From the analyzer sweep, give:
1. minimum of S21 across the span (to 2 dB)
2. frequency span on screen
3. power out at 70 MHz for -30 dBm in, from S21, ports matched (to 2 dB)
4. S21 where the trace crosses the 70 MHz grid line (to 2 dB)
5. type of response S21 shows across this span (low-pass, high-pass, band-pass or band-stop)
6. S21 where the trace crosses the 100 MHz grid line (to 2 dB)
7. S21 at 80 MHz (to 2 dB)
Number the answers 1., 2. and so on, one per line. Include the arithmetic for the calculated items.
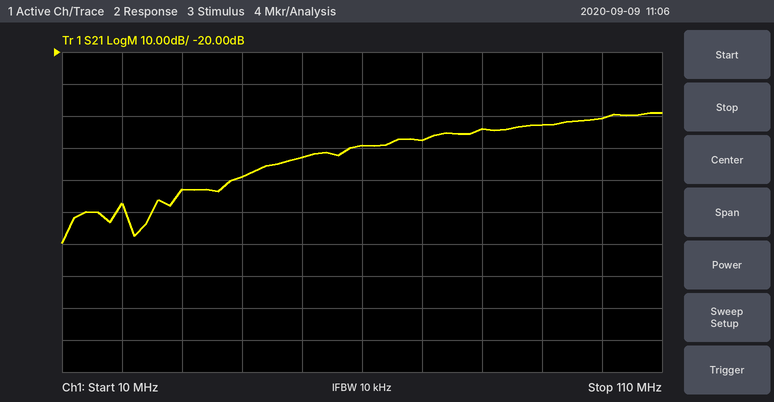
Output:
1. -80 dB
2. 100 MHz
3. -30 dBm + (-48 dB) = -78 dBm
4. -48 dB
5. high-pass
6. -40 dB
7. -44 dB
